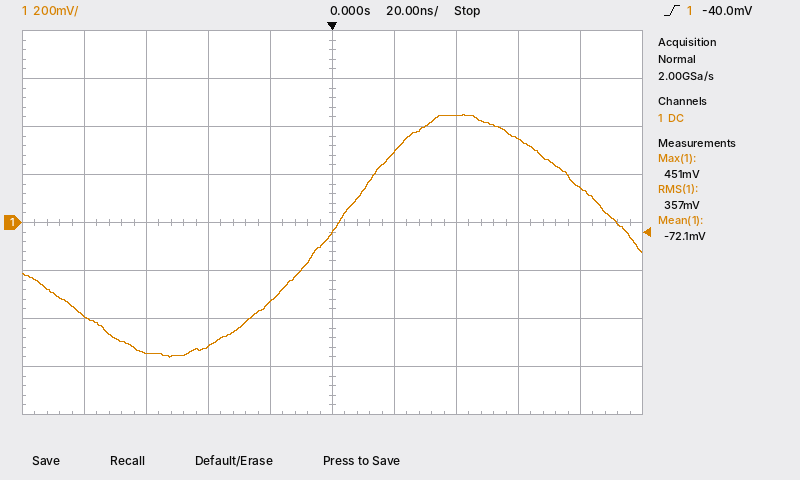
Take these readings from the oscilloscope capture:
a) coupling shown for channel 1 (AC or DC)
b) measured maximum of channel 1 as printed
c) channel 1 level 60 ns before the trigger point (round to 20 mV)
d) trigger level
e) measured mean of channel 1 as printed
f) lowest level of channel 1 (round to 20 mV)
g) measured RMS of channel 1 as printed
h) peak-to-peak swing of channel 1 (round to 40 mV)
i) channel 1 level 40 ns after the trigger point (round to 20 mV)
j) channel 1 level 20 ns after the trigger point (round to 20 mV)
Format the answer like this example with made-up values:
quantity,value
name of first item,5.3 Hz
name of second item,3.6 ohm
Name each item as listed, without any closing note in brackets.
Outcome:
quantity,value
coupling shown for channel 1,DC
measured maximum of channel 1 as printed,451 mV
channel 1 level 60 ns before the trigger point,-540 mV
trigger level,-40.0 mV
measured mean of channel 1 as printed,-72.1 mV
lowest level of channel 1,-560 mV
measured RMS of channel 1 as printed,357 mV
peak-to-peak swing of channel 1,1.00 V
channel 1 level 40 ns after the trigger point,440 mV
channel 1 level 20 ns after the trigger point,300 mV
